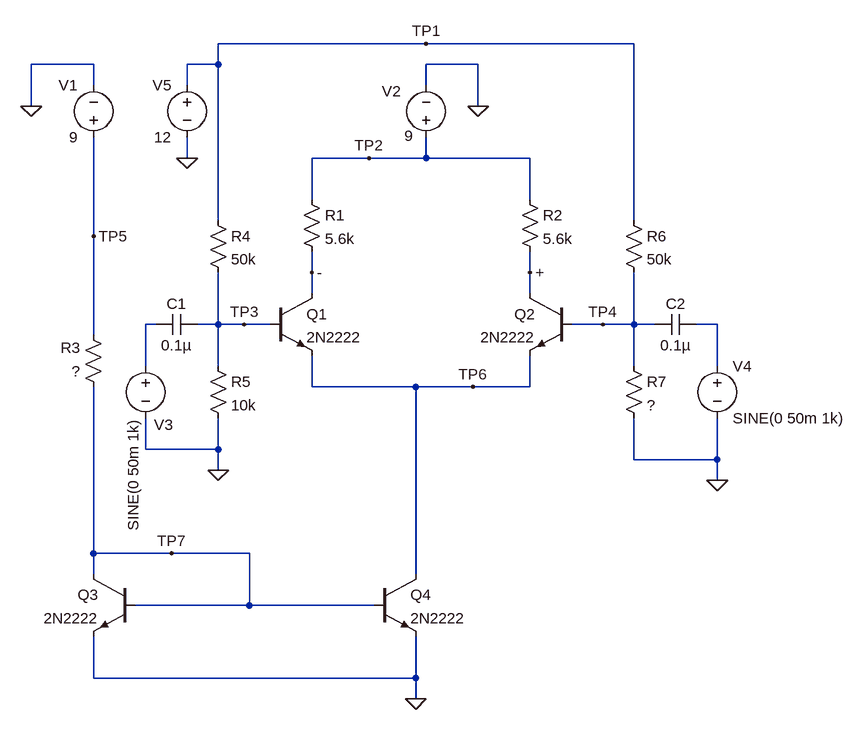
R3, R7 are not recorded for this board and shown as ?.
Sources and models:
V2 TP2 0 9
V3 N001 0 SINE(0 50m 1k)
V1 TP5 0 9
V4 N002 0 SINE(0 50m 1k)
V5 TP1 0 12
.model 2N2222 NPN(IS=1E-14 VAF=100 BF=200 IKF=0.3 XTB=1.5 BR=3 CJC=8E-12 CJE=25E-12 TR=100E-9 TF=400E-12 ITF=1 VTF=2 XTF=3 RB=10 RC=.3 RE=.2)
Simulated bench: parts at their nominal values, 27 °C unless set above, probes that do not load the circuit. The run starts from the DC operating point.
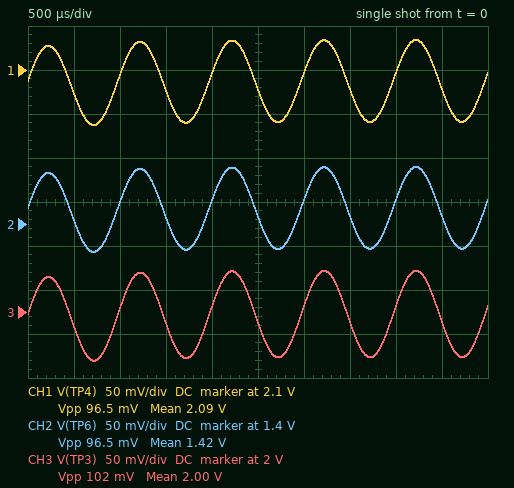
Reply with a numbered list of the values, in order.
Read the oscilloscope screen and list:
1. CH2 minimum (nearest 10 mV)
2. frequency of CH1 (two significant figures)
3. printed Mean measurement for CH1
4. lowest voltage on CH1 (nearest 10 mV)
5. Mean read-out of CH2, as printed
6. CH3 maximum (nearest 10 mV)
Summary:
1. 1.37 V
2. 1.0 kHz
3. 2.09 V
4. 2.04 V
5. 1.42 V
6. 2.05 V
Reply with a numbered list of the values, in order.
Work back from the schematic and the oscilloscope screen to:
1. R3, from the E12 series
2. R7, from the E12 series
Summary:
1. 5.6 kΩ
2. 18 kΩ
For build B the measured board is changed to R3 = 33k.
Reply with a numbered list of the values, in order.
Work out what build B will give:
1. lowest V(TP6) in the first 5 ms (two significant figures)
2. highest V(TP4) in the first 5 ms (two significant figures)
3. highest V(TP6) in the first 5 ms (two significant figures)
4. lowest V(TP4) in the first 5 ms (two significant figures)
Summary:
1. 2.5 V
2. 3.2 V
3. 2.6 V
4. 3.1 V
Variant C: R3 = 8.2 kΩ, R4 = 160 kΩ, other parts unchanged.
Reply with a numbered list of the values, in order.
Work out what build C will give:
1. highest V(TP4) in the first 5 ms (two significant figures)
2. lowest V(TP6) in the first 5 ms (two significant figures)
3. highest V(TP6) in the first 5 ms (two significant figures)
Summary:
1. 3.2 V
2. 2.4 V
3. 2.5 V
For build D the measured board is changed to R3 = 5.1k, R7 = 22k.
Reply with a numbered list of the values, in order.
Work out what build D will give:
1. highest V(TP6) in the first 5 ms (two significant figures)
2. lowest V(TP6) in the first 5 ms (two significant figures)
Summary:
1. 1.4 V
2. 1.3 V
